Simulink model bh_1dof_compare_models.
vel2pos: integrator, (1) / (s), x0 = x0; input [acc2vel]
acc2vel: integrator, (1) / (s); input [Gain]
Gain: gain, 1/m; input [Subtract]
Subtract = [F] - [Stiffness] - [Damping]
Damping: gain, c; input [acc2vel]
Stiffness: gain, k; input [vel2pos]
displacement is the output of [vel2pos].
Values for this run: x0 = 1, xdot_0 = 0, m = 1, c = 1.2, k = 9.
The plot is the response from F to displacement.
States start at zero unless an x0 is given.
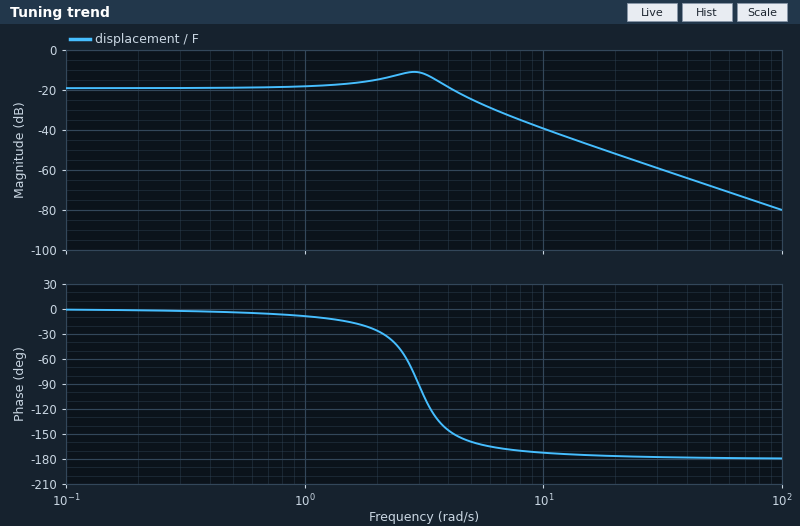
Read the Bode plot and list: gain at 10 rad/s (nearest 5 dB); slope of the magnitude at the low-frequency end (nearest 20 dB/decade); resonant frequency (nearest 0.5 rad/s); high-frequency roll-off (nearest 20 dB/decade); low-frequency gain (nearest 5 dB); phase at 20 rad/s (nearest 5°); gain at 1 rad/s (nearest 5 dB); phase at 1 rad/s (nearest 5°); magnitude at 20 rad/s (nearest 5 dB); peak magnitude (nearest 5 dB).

-40 dB
0 dB/decade
3.0 rad/s
-40 dB/decade
-20 dB
-175°
-20 dB
-10°
-50 dB
-10 dB
